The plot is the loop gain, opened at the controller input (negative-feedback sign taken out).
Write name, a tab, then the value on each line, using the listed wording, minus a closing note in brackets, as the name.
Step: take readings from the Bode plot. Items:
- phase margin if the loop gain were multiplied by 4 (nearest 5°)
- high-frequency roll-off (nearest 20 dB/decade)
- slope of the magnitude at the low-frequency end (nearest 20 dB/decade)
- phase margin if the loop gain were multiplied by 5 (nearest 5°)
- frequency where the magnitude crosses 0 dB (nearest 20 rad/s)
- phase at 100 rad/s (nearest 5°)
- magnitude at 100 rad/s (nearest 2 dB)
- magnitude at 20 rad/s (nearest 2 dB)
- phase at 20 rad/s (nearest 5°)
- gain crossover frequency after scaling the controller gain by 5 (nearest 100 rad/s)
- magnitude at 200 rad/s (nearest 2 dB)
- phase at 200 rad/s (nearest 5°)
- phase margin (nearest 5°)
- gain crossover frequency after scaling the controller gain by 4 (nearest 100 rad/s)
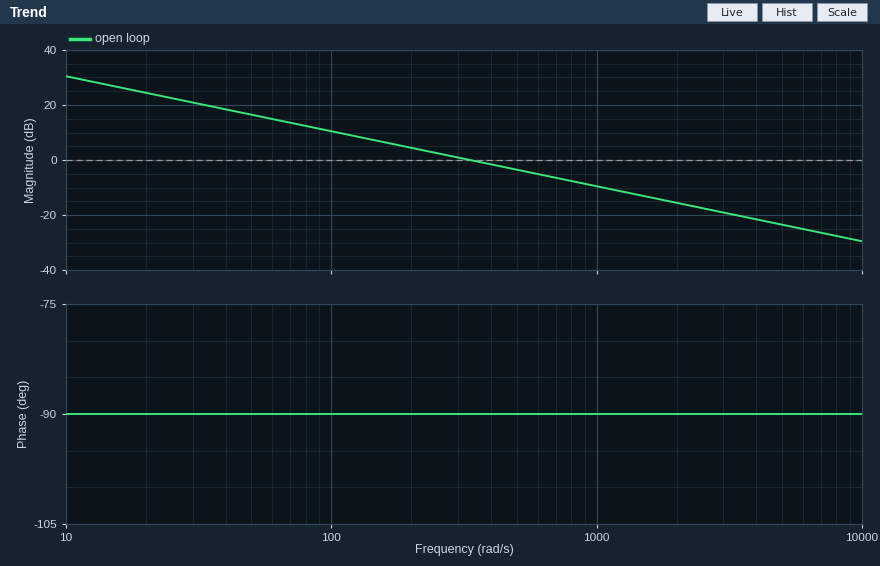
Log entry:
phase margin if the loop gain were multiplied by 4	90°
high-frequency roll-off	-20 dB/decade
slope of the magnitude at the low-frequency end	-20 dB/decade
phase margin if the loop gain were multiplied by 5	90°
frequency where the magnitude crosses 0 dB	340 rad/s
phase at 100 rad/s	-90°
magnitude at 100 rad/s	10 dB
magnitude at 20 rad/s	24 dB
phase at 20 rad/s	-90°
gain crossover frequency after scaling the controller gain by 5	1700 rad/s
magnitude at 200 rad/s	4 dB
phase at 200 rad/s	-90°
phase margin	90°
gain crossover frequency after scaling the controller gain by 4	1300 rad/s
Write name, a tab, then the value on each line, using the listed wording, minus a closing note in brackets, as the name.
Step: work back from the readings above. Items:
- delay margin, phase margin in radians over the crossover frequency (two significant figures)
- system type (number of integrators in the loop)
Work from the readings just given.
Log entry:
delay margin, phase margin in radians over the crossover frequency	0.0046 s
system type	1
